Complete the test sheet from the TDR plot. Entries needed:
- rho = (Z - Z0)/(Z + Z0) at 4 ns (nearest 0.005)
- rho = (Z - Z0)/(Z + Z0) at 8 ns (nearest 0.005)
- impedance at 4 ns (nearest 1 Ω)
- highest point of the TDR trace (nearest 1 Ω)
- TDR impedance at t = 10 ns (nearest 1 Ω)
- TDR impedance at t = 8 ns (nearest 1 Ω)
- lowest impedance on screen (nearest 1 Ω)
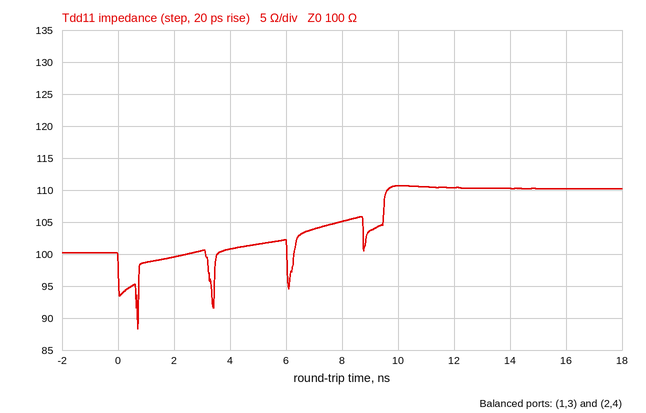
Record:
+0.005
+0.025
101 Ω
111 Ω
111 Ω
105 Ω
88 Ω
